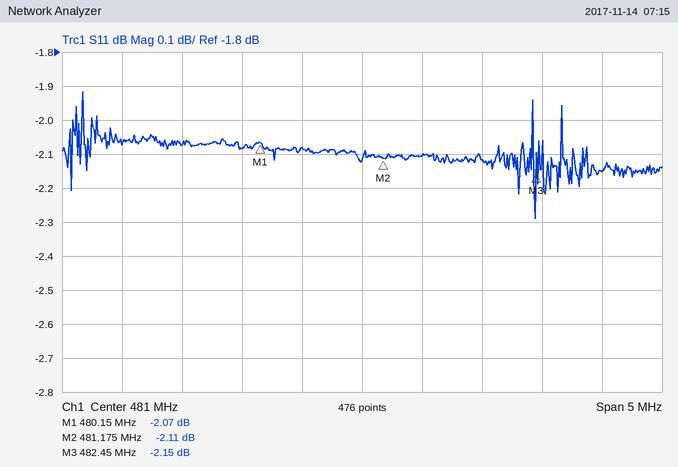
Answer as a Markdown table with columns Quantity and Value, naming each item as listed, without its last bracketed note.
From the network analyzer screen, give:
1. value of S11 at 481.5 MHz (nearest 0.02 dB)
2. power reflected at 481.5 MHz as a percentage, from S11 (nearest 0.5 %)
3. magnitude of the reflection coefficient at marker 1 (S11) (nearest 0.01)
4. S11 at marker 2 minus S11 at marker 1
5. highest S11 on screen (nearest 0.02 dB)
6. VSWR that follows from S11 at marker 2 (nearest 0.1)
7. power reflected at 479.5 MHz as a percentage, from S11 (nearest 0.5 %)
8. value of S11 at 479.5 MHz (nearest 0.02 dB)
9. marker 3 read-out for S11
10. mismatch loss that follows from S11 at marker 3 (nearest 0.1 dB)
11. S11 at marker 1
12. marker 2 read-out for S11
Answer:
| Quantity | Value |
|---|---|
| value of S11 at 481.5 MHz | -2.10 dB |
| power reflected at 481.5 MHz as a percentage, from S11 | 61.5 % |
| magnitude of the reflection coefficient at marker 1 (S11) | 0.79 |
| S11 at marker 2 minus S11 at marker 1 | -0.04 dB |
| highest S11 on screen | -1.92 dB |
| VSWR that follows from S11 at marker 2 | 8.3 |
| power reflected at 479.5 MHz as a percentage, from S11 | 62.0 % |
| value of S11 at 479.5 MHz | -2.08 dB |
| marker 3 read-out for S11 | -2.15 dB |
| mismatch loss that follows from S11 at marker 3 | 4.1 dB |
| S11 at marker 1 | -2.07 dB |
| marker 2 read-out for S11 | -2.11 dB |
